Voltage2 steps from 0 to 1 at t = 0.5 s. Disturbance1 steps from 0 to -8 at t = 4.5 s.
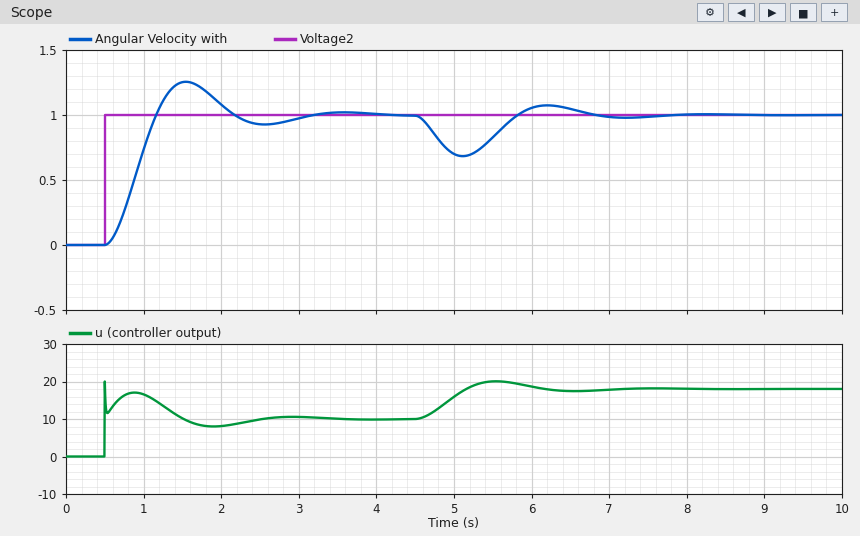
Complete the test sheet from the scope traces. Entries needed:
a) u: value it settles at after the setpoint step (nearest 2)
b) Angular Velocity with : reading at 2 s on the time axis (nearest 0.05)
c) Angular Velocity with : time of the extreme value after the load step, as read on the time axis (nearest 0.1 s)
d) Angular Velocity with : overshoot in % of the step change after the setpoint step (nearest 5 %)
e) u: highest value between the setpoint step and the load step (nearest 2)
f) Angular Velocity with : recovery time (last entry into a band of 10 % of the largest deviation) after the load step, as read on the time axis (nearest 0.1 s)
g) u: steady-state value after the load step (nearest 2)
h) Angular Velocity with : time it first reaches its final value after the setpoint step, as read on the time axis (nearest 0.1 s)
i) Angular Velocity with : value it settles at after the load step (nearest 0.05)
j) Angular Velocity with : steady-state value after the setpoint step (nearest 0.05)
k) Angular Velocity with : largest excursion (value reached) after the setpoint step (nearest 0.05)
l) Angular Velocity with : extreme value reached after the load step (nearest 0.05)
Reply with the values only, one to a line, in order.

10
1.10
5.1 s
25 %
20
6.6 s
18
1.2 s
1.00
1.00
1.25
0.70
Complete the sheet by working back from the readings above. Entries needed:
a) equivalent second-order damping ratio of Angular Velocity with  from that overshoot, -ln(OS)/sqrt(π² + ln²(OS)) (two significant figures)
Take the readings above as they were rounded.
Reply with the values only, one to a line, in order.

0.40
